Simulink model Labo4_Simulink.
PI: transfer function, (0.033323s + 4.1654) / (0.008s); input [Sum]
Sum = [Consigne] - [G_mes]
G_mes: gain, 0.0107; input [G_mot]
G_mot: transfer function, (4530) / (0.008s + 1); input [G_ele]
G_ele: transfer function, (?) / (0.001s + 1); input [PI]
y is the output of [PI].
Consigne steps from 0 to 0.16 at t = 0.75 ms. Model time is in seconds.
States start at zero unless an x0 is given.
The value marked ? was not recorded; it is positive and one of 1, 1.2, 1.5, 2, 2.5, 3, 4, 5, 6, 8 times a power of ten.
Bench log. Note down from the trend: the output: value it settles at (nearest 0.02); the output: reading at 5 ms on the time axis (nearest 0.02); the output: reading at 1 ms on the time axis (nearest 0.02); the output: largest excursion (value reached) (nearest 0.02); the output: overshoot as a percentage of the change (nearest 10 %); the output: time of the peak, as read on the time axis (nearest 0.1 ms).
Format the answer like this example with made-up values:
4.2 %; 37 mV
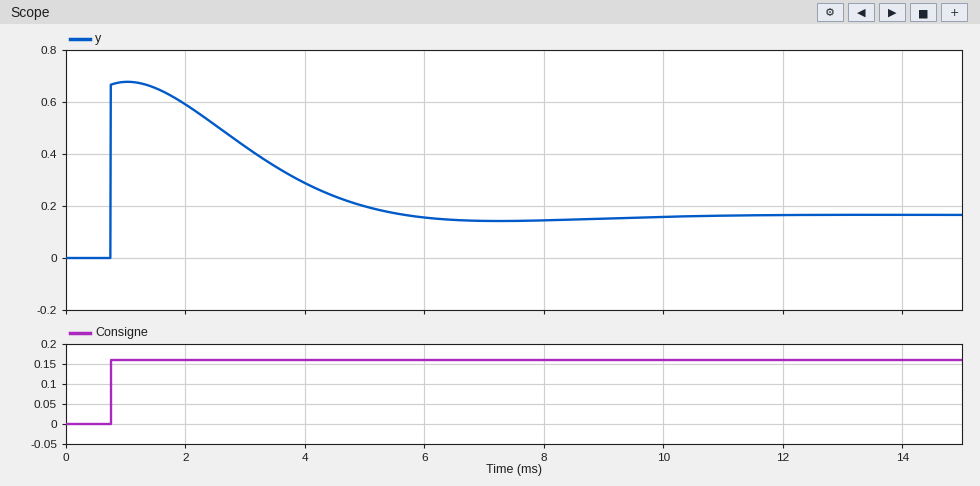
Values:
0.16; 0.20; 0.68; 0.68; 310 %; 1.0 ms
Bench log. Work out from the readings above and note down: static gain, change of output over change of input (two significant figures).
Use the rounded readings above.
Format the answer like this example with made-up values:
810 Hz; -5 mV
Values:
1.0
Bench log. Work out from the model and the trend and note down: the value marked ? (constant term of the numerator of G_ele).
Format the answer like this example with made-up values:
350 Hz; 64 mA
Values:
0.02
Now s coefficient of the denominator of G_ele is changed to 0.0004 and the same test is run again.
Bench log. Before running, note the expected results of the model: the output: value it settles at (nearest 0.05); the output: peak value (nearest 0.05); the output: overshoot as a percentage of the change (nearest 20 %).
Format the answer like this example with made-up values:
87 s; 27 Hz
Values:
0.15; 0.65; 300 %
